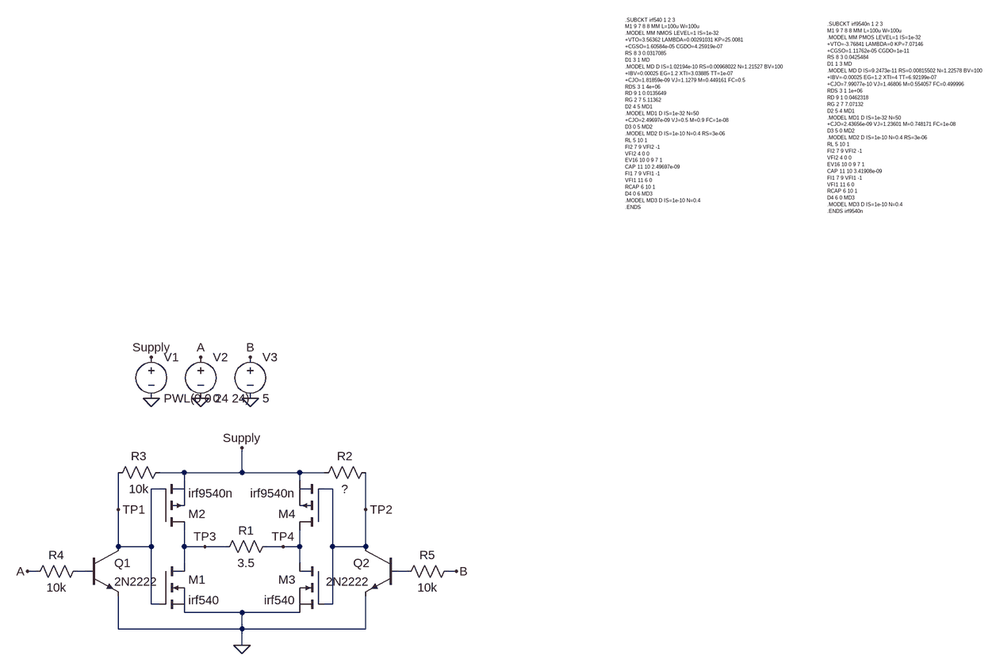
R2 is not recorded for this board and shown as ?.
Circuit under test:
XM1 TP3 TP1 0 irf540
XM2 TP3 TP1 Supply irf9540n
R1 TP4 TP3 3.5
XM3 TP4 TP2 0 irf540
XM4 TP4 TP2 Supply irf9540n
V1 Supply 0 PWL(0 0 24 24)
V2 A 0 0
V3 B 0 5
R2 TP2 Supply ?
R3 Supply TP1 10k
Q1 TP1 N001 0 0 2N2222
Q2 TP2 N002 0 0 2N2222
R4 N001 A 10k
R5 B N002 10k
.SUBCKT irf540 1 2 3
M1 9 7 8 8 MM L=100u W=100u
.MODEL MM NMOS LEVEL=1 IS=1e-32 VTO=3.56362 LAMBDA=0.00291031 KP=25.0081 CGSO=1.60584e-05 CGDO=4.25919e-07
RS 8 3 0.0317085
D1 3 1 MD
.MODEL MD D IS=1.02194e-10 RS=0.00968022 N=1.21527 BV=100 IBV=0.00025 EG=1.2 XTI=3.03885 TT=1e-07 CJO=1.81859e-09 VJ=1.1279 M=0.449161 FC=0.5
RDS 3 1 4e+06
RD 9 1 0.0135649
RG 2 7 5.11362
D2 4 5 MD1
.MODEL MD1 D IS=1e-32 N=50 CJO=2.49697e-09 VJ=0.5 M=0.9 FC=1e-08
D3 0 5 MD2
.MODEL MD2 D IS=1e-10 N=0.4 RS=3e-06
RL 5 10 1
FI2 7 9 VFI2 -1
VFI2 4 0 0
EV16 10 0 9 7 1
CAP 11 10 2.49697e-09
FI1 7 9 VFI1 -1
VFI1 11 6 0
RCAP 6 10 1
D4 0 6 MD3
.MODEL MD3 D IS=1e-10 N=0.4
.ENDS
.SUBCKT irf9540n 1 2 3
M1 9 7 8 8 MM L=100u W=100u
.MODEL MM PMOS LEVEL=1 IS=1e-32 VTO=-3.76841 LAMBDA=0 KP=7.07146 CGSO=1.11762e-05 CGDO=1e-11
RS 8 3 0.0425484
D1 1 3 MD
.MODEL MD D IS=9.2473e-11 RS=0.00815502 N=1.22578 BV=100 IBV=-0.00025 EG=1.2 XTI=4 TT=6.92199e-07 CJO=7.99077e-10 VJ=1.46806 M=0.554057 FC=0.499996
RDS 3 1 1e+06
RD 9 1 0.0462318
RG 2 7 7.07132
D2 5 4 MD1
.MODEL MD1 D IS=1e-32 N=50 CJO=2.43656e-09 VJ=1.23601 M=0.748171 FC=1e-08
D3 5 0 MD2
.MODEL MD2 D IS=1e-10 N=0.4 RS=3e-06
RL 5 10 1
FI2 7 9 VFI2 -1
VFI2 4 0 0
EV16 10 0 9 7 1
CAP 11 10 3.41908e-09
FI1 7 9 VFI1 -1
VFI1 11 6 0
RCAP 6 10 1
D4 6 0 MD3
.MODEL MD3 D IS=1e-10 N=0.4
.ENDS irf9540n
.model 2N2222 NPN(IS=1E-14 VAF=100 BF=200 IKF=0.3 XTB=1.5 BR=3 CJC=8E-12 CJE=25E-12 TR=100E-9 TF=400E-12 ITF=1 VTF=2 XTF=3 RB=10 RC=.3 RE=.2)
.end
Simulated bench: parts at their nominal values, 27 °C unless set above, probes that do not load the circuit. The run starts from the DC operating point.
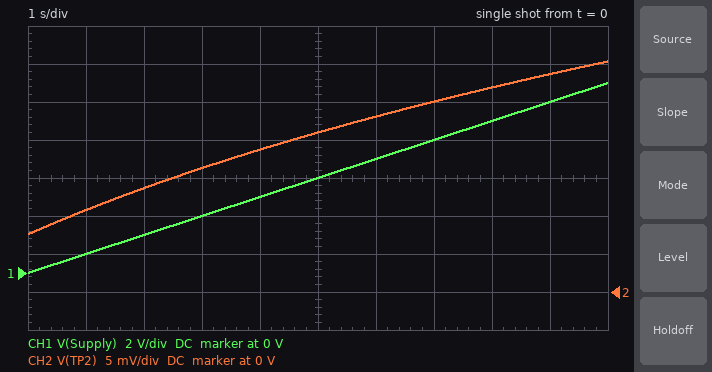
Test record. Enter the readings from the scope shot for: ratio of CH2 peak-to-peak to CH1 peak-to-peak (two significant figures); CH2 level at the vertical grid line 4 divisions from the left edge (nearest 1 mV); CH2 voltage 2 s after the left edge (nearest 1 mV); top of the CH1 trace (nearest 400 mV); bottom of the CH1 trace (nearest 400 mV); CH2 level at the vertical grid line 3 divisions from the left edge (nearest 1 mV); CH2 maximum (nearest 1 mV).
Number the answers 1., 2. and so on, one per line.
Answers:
1. 0.0023
2. 19 mV
3. 14 mV
4. 10.0 V
5. 0 V
6. 16 mV
7. 30 mV
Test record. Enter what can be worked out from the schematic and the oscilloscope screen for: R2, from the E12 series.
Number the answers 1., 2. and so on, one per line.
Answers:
1. 4.7 kΩ
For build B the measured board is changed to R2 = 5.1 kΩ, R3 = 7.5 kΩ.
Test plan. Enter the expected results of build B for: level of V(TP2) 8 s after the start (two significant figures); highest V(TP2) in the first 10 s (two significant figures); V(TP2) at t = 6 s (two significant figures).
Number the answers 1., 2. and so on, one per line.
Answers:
1. 26 mV
2. 29 mV
3. 22 mV
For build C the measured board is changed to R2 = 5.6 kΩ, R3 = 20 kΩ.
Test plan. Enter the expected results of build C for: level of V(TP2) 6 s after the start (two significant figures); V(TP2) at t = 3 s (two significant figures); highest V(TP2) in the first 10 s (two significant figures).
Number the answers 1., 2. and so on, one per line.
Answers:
1. 21 mV
2. 15 mV
3. 28 mV
